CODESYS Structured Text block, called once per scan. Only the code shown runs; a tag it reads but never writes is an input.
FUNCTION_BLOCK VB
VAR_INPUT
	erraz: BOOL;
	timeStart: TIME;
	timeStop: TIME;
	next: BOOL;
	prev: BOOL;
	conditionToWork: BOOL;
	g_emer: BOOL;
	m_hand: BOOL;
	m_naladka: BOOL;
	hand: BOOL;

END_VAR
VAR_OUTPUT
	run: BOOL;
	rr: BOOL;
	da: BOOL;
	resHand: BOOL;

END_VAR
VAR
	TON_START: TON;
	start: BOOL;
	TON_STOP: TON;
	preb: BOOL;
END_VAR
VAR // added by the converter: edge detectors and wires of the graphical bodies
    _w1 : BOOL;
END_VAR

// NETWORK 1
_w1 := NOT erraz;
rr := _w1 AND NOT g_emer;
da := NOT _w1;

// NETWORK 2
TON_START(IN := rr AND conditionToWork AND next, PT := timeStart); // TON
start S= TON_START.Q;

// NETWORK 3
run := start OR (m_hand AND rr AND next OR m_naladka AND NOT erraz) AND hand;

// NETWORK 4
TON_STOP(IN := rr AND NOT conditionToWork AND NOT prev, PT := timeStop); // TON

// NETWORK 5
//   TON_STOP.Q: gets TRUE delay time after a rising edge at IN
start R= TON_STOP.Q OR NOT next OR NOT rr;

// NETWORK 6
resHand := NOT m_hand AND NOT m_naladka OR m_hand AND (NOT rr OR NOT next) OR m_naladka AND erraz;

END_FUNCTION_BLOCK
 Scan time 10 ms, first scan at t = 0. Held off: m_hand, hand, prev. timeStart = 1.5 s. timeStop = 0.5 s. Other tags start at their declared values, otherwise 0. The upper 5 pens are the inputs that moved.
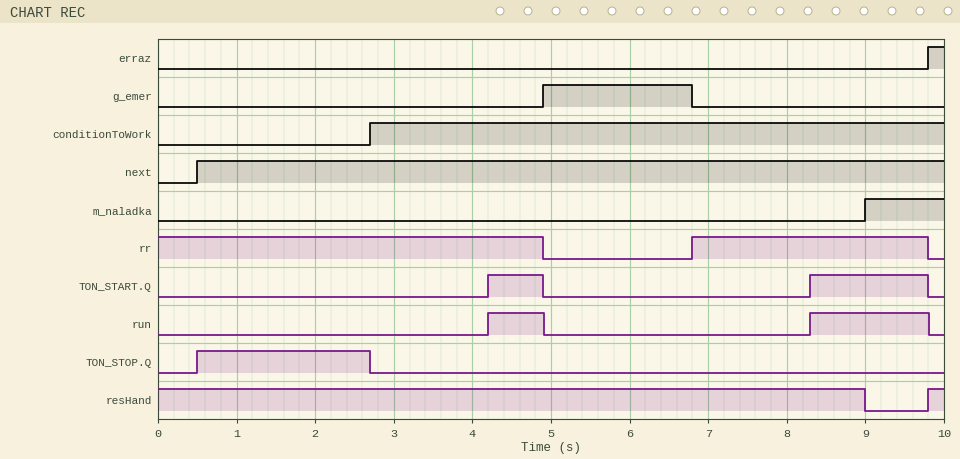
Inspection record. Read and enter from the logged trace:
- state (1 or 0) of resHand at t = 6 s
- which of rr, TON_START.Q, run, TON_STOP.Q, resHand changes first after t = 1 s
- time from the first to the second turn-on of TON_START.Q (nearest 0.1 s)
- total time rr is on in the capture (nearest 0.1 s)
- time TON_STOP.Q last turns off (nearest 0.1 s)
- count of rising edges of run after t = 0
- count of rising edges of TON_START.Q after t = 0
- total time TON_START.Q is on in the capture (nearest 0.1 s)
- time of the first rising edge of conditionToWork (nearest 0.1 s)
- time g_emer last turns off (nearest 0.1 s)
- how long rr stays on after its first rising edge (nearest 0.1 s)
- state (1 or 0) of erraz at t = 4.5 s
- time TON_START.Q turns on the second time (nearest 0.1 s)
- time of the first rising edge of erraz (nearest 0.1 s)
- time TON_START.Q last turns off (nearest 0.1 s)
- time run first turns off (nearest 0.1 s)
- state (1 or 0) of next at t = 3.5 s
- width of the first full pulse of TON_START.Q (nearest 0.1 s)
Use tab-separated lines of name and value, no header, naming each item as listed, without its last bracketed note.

state (1 or 0) of resHand at t = 6 s	1
which of rr, TON_START.Q, run, TON_STOP.Q, resHand changes first after t = 1 s	TON_STOP.Q
time from the first to the second turn-on of TON_START.Q	4.1 s
total time rr is on in the capture	7.9 s
time TON_STOP.Q last turns off	2.7 s
count of rising edges of run after t = 0	2
count of rising edges of TON_START.Q after t = 0	2
total time TON_START.Q is on in the capture	2.2 s
time of the first rising edge of conditionToWork	2.7 s
time g_emer last turns off	6.8 s
how long rr stays on after its first rising edge	3.0 s
state (1 or 0) of erraz at t = 4.5 s	0
time TON_START.Q turns on the second time	8.3 s
time of the first rising edge of erraz	9.8 s
time TON_START.Q last turns off	9.8 s
time run first turns off	4.9 s
state (1 or 0) of next at t = 3.5 s	1
width of the first full pulse of TON_START.Q	0.7 s
